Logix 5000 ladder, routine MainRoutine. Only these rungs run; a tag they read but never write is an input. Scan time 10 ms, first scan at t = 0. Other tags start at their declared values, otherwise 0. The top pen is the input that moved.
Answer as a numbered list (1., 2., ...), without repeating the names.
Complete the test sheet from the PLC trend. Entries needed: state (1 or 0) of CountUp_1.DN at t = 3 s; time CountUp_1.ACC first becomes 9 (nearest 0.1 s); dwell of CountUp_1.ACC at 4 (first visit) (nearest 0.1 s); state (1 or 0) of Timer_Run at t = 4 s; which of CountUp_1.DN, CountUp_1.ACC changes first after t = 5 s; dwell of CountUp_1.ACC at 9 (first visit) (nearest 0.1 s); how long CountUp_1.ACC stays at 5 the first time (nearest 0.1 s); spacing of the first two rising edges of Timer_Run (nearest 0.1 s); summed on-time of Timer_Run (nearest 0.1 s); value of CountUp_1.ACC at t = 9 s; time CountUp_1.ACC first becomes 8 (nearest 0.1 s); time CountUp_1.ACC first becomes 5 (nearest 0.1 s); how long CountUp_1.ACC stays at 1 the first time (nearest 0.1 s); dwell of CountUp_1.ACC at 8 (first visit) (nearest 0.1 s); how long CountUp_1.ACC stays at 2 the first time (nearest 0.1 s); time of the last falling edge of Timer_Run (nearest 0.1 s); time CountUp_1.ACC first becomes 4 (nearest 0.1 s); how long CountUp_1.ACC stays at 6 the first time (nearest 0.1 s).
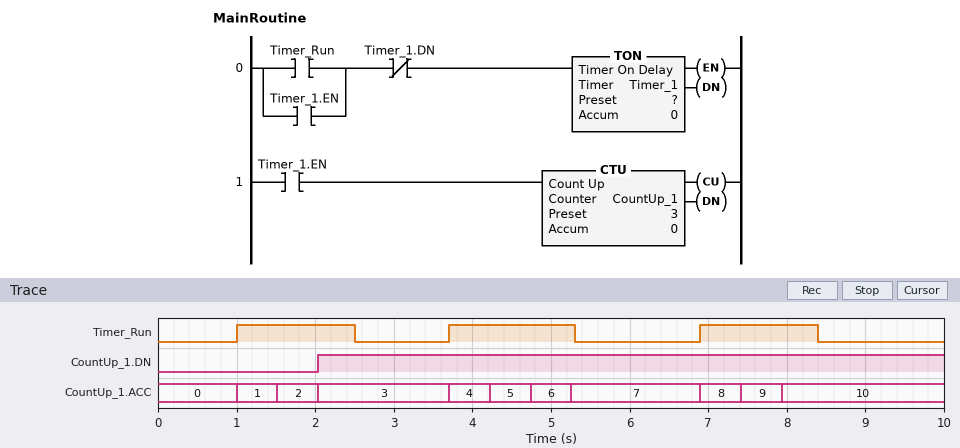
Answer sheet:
1. 1
2. 7.4 s
3. 0.5 s
4. 1
5. CountUp_1.ACC
6. 0.5 s
7. 0.5 s
8. 2.7 s
9. 4.6 s
10. 10
11. 6.9 s
12. 4.2 s
13. 0.5 s
14. 0.5 s
15. 0.5 s
16. 8.4 s
17. 3.7 s
18. 0.5 s
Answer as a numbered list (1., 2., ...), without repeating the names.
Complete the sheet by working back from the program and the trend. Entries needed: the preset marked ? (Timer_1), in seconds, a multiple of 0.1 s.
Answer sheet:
1. 0.5 s
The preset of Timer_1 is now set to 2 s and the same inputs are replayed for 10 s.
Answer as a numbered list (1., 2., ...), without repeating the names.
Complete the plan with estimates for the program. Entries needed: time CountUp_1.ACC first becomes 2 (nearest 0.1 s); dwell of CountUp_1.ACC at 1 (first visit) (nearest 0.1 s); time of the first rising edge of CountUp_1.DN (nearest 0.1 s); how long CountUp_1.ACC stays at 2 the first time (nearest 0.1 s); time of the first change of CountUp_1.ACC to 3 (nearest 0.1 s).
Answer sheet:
1. 3.7 s
2. 2.7 s
3. 6.9 s
4. 3.2 s
5. 6.9 s
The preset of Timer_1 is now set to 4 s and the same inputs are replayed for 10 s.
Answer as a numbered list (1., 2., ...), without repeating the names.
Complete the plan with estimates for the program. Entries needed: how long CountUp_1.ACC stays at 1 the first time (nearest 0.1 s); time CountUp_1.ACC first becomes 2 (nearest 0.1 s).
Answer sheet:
1. 4.0 s
2. 5.0 s
